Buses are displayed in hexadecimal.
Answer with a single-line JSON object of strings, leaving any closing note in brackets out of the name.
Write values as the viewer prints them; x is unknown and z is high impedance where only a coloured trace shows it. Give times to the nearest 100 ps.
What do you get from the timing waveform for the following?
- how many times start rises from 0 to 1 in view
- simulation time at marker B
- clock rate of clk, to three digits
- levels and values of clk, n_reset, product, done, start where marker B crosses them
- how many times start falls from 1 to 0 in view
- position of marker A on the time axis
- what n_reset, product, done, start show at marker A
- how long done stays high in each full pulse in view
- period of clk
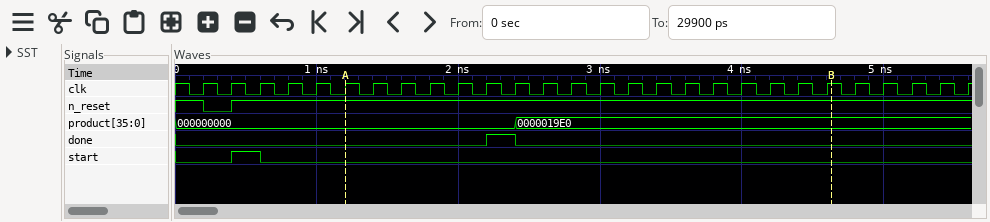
{"how many times start rises from 0 to 1 in view": "1", "simulation time at marker B": "4600 ps", "clock rate of clk, to three digits": "5.00 GHz", "levels and values of clk, n_reset, product, done, start where marker B crosses them": "clk=1, n_reset=1, product=0000019E0, done=0, start=0", "how many times start falls from 1 to 0 in view": "1", "position of marker A on the time axis": "1200 ps", "what n_reset, product, done, start show at marker A": "n_reset=1, product=000000000, done=0, start=0", "how long done stays high in each full pulse in view": "200 ps", "period of clk": "200 ps"}
